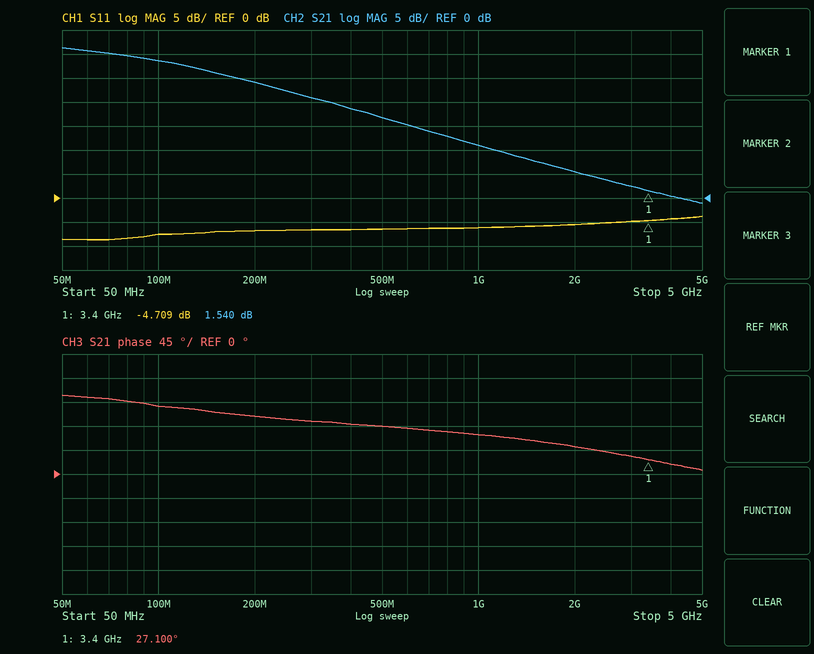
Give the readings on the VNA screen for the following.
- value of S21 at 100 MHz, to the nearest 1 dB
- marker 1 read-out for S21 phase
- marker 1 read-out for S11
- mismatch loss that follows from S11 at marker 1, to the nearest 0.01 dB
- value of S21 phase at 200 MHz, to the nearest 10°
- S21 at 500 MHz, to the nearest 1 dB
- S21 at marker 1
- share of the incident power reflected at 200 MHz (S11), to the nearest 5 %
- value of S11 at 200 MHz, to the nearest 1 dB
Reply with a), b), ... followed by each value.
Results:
a) 29 dB
b) 27.100°
c) -4.709 dB
d) 1.79 dB
e) 110°
f) 17 dB
g) 1.540 dB
h) 20 %
i) -7 dB
